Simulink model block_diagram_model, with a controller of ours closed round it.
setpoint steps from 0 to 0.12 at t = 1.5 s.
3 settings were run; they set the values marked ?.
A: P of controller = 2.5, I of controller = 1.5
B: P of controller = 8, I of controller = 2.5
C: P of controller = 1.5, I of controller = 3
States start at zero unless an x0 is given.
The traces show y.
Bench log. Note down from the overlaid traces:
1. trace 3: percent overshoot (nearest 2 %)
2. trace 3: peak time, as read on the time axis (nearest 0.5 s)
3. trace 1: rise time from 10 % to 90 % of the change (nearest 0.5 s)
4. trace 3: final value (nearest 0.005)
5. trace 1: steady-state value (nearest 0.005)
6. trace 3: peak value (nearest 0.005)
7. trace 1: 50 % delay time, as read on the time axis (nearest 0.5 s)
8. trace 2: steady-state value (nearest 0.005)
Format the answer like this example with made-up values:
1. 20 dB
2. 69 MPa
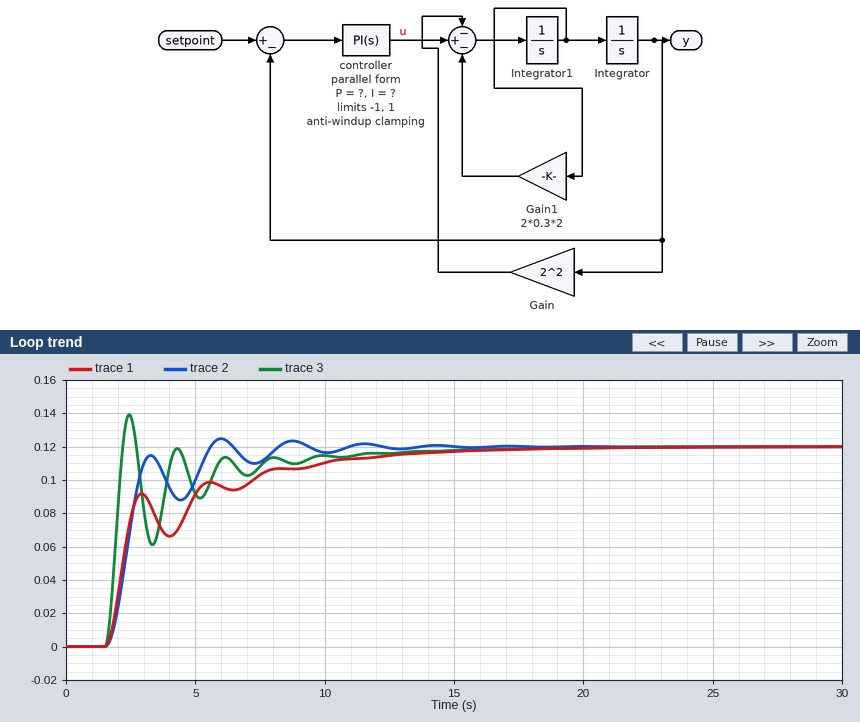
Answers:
1. 16 %
2. 2.5 s
3. 7.5 s
4. 0.120
5. 0.120
6. 0.140
7. 2.5 s
8. 0.120
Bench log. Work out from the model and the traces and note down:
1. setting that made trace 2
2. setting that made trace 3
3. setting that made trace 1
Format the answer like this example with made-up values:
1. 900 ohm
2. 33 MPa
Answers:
1. C
2. B
3. A
